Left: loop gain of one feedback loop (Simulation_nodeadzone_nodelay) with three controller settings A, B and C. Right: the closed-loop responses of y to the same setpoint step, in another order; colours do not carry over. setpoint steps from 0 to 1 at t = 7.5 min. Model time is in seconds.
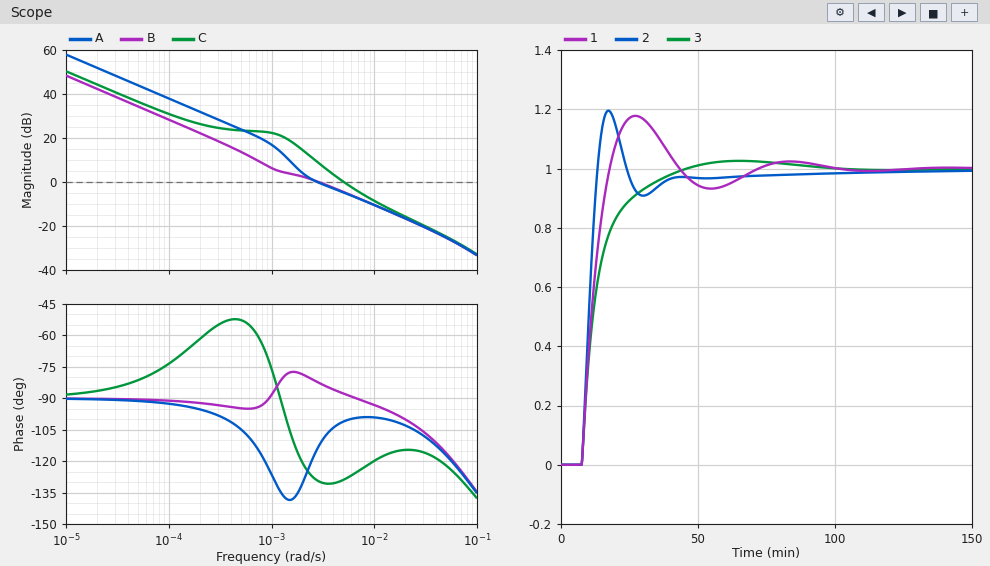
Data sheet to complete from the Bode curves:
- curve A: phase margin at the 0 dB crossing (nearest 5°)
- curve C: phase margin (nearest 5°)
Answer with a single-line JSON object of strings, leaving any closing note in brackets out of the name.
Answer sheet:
{"curve A: phase margin at the 0 dB crossing": "65°", "curve C: phase margin": "50°"}
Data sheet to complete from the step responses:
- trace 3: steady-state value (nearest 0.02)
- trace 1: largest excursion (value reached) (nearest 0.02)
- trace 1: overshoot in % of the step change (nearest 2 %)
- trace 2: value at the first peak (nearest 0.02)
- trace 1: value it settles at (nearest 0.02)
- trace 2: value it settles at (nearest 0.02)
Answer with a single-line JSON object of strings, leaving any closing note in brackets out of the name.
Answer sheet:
{"trace 3: steady-state value": "1.00", "trace 1: largest excursion (value reached)": "1.18", "trace 1: overshoot in % of the step change": "18 %", "trace 2: value at the first peak": "1.20", "trace 1: value it settles at": "1.00", "trace 2: value it settles at": "1.00"}
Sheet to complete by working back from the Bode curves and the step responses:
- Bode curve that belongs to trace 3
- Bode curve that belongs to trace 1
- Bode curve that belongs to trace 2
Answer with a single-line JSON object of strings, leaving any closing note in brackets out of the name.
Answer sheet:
{"Bode curve that belongs to trace 3": "B", "Bode curve that belongs to trace 1": "A", "Bode curve that belongs to trace 2": "C"}
